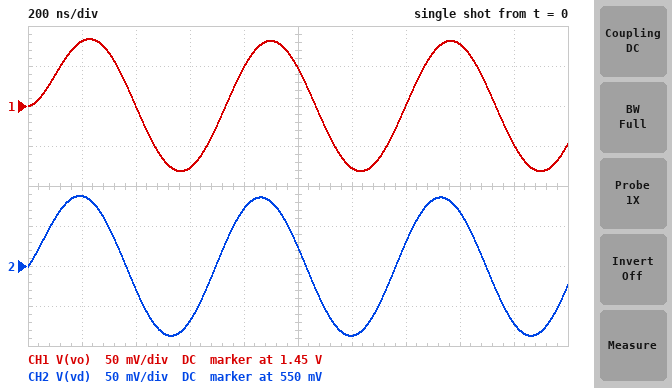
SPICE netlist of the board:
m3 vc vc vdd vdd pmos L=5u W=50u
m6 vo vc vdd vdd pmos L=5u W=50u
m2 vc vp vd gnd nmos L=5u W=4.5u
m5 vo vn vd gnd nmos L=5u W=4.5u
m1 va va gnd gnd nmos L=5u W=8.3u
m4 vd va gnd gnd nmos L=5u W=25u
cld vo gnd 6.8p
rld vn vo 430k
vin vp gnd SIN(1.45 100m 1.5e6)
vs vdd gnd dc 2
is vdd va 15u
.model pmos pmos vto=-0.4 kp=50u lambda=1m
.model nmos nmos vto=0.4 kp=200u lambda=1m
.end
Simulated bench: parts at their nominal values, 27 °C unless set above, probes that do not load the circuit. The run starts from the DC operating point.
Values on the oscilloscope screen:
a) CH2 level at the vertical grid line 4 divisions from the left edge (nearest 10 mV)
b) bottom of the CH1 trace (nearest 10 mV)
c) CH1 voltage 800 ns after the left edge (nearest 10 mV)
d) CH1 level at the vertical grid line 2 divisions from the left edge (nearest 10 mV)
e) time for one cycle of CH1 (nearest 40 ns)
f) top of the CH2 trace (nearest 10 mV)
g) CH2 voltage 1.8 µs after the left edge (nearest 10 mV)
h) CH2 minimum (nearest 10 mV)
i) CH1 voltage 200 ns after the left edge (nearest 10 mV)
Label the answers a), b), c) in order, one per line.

a) 620 mV
b) 1.37 V
c) 1.50 V
d) 1.45 V
e) 680 ns
f) 640 mV
g) 480 mV
h) 460 mV
i) 1.53 V
